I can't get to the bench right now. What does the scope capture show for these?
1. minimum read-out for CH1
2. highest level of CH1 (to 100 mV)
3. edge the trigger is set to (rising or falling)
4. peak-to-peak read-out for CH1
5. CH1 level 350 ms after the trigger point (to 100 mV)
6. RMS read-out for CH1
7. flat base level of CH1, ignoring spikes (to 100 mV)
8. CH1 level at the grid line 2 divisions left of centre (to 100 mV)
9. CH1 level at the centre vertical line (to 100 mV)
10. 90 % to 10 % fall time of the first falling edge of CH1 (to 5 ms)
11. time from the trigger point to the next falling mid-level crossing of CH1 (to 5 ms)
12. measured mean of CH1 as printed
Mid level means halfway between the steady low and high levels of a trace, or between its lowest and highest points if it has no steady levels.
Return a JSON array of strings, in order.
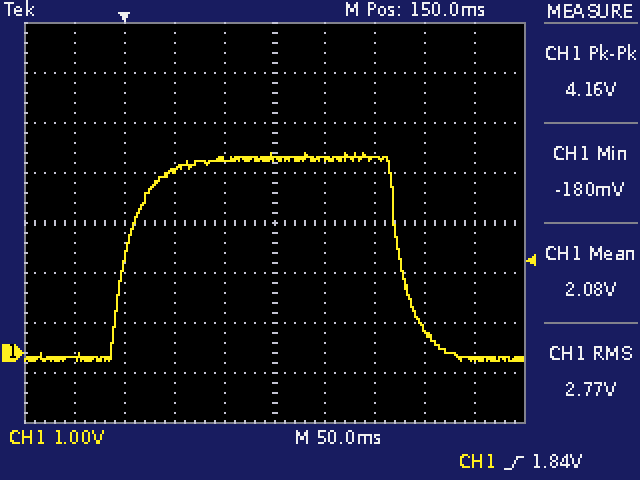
["-180 mV", "4.0 V", "rising", "4.16 V", "-100 mV", "2.77 V", "-100 mV", "3.7 V", "3.9 V", "40 ms", "275 ms", "2.08 V"]
